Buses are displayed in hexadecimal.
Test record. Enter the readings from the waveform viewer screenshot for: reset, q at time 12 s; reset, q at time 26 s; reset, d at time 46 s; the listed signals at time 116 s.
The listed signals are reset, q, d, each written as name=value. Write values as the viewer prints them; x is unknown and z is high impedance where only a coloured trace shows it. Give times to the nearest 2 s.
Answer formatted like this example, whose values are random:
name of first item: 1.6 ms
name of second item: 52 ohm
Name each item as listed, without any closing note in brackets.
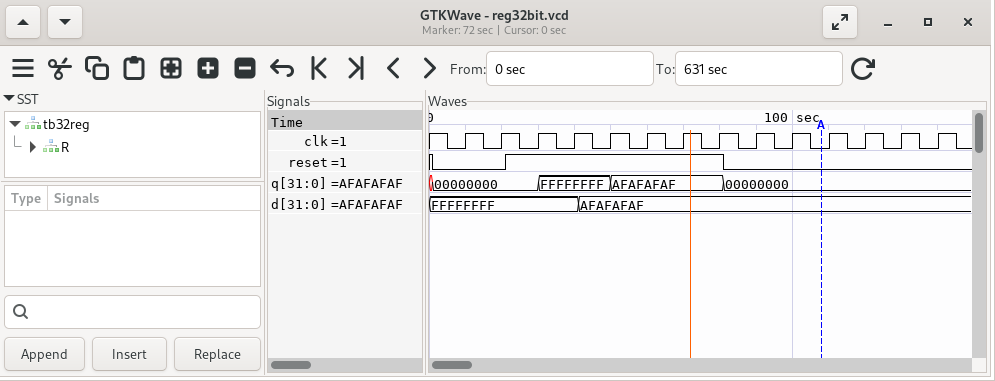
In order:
reset, q at time 12 s: reset=0, q=00000000
reset, q at time 26 s: reset=1, q=00000000
reset, d at time 46 s: reset=1, d=AFAFAFAF
the listed signals at time 116 s: reset=0, q=00000000, d=AFAFAFAF
